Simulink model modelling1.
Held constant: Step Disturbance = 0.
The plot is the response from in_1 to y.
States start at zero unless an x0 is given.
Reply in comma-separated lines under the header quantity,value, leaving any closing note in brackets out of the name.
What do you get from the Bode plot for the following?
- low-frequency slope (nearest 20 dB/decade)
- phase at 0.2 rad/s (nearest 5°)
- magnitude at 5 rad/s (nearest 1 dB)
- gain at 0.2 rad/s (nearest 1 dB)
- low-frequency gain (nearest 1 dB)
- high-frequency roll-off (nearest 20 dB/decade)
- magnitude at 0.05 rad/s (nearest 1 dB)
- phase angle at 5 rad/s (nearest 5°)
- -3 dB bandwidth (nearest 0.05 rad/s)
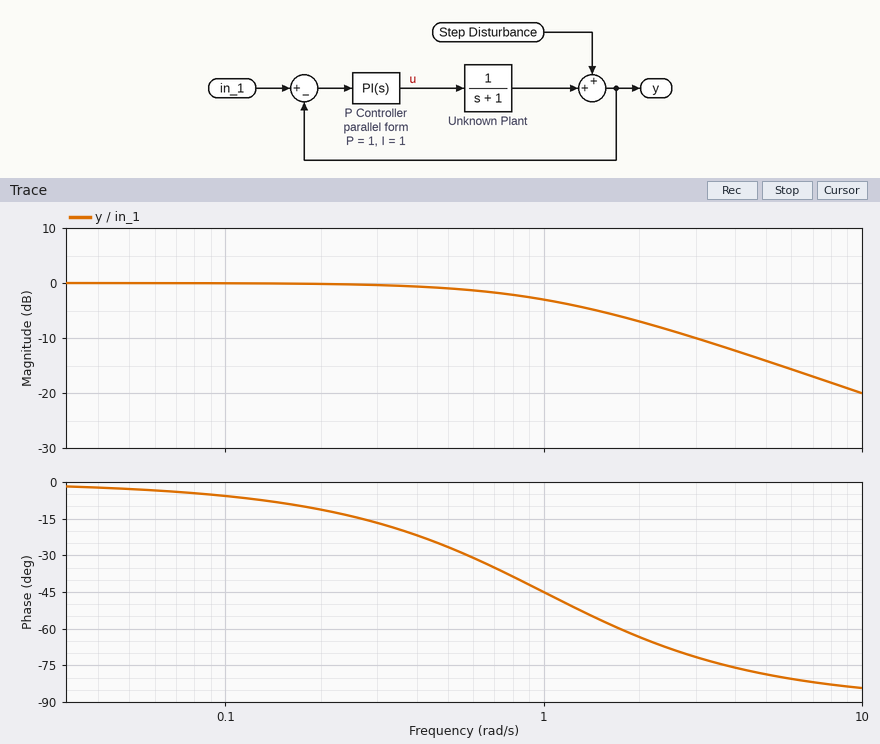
quantity,value
low-frequency slope,0 dB/decade
phase at 0.2 rad/s,-10°
magnitude at 5 rad/s,-14 dB
gain at 0.2 rad/s,0 dB
low-frequency gain,0 dB
high-frequency roll-off,-20 dB/decade
magnitude at 0.05 rad/s,0 dB
phase angle at 5 rad/s,-80°
-3 dB bandwidth,1.00 rad/s
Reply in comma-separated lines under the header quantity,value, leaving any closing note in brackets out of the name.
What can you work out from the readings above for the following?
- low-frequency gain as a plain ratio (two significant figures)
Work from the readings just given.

quantity,value
low-frequency gain as a plain ratio,1.0
